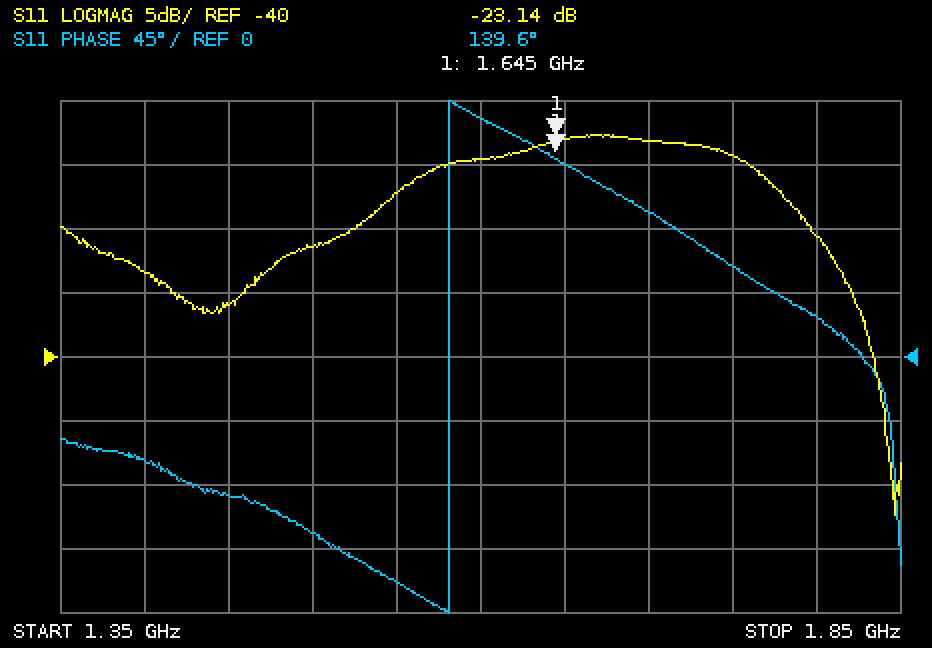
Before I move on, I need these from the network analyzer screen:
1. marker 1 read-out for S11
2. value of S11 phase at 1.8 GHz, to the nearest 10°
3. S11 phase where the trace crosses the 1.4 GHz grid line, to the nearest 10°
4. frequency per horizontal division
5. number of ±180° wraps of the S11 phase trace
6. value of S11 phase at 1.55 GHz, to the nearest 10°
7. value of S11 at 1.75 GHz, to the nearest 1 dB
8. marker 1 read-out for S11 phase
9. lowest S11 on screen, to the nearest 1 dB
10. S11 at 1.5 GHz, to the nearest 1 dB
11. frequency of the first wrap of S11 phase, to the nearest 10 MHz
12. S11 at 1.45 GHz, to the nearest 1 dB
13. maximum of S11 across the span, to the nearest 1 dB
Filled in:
-23.14 dB
30°
-70°
50 MHz
1
-160°
-24 dB
139.6°
-52 dB
-31 dB
1.58 GHz
-36 dB
-23 dB
